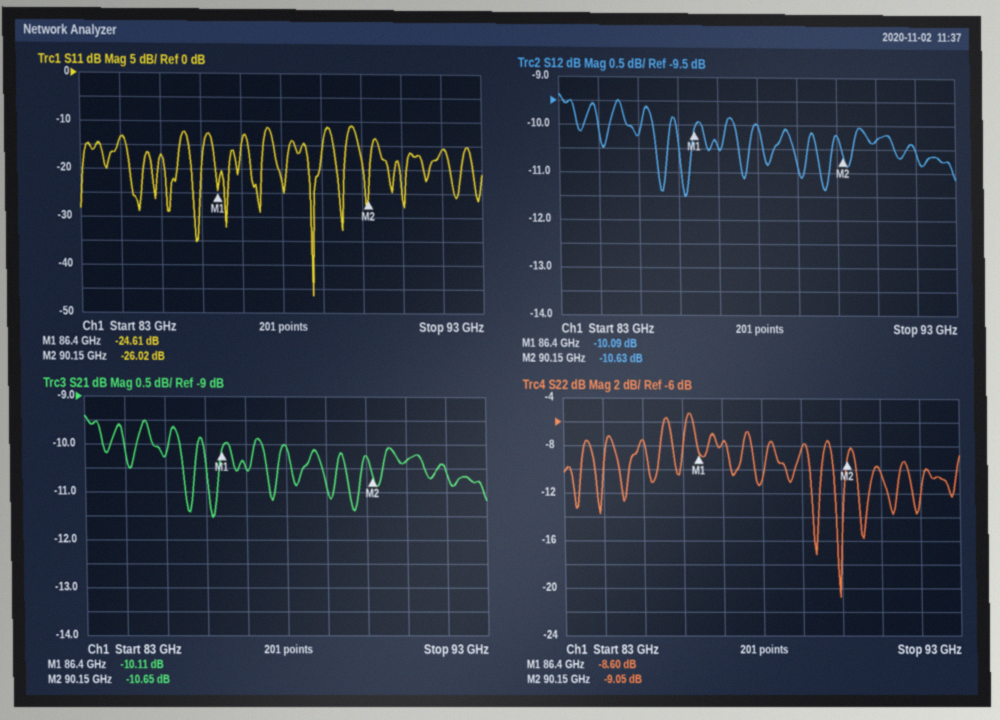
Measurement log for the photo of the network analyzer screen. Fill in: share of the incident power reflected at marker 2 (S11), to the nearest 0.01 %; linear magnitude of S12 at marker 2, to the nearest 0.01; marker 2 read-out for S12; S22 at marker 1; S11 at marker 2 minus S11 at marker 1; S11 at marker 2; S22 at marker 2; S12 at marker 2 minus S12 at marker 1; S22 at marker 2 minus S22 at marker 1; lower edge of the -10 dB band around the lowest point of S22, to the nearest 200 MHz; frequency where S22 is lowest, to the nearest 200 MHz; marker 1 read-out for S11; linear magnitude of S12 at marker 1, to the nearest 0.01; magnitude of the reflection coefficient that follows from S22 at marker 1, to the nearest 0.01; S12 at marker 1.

0.25 %
0.29
-10.63 dB
-8.60 dB
-1.41 dB
-26.02 dB
-9.05 dB
-0.54 dB
-0.45 dB
89.8 GHz
90.0 GHz
-24.61 dB
0.31
0.37
-10.09 dB
